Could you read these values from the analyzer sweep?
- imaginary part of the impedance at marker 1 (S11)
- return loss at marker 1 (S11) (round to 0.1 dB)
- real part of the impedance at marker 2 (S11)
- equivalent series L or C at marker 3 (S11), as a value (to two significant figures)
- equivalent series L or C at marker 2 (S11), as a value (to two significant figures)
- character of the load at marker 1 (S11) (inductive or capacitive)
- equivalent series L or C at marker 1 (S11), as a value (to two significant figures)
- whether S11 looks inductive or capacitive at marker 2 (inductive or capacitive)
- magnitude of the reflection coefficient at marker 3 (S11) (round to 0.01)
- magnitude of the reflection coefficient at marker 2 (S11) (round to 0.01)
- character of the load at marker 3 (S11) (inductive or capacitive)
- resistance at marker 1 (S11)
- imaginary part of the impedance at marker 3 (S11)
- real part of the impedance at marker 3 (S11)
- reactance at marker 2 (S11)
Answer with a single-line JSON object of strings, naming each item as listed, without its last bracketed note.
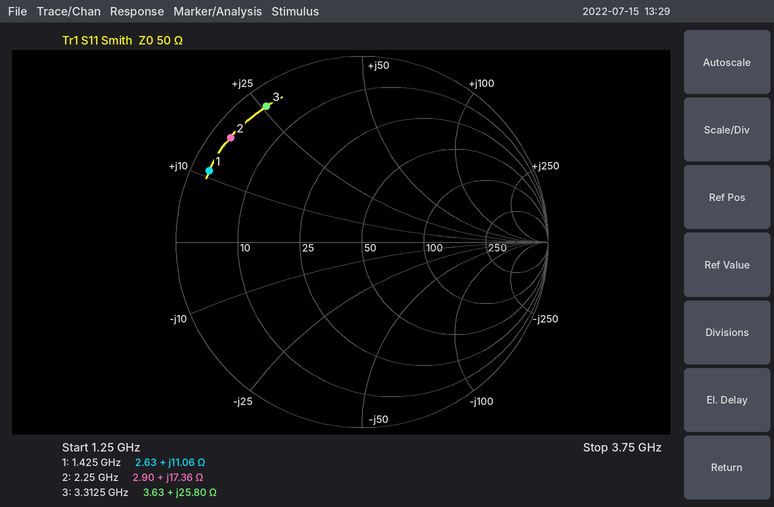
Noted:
{"imaginary part of the impedance at marker 1": "+11.06 Ω", "return loss at marker 1 (S11)": "0.9 dB", "real part of the impedance at marker 2": "2.90 Ω", "equivalent series L or C at marker 3 (S11), as a value": "1.2 nH", "equivalent series L or C at marker 2 (S11), as a value": "1.2 nH", "character of the load at marker 1 (S11)": "inductive", "equivalent series L or C at marker 1 (S11), as a value": "1.2 nH", "whether S11 looks inductive or capacitive at marker 2": "inductive", "magnitude of the reflection coefficient at marker 3 (S11)": "0.89", "magnitude of the reflection coefficient at marker 2 (S11)": "0.90", "character of the load at marker 3 (S11)": "inductive", "resistance at marker 1": "2.63 Ω", "imaginary part of the impedance at marker 3": "+25.80 Ω", "real part of the impedance at marker 3": "3.63 Ω", "reactance at marker 2": "+17.36 Ω"}
